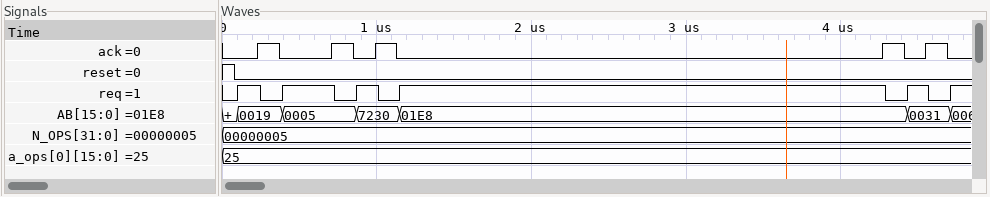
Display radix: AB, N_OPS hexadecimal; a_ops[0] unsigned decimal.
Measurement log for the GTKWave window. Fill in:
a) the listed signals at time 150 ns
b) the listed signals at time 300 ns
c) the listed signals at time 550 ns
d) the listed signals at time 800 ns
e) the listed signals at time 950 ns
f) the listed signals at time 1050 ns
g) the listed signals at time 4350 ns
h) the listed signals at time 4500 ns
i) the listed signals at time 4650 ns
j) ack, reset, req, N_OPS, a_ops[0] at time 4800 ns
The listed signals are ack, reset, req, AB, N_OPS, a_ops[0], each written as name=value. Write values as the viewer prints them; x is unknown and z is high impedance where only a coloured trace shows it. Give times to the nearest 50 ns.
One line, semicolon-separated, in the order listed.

ack=0, reset=0, req=1, AB=0019, N_OPS=00000005, a_ops[0]=25; ack=1, reset=0, req=0, AB=0019, N_OPS=00000005, a_ops[0]=25; ack=0, reset=0, req=1, AB=0005, N_OPS=00000005, a_ops[0]=25; ack=1, reset=0, req=0, AB=0005, N_OPS=00000005, a_ops[0]=25; ack=0, reset=0, req=1, AB=7230, N_OPS=00000005, a_ops[0]=25; ack=1, reset=0, req=0, AB=7230, N_OPS=00000005, a_ops[0]=25; ack=1, reset=0, req=0, AB=01E8, N_OPS=00000005, a_ops[0]=25; ack=0, reset=0, req=1, AB=0031, N_OPS=00000005, a_ops[0]=25; ack=1, reset=0, req=0, AB=0031, N_OPS=00000005, a_ops[0]=25; ack=0, reset=0, req=1, N_OPS=00000005, a_ops[0]=25
